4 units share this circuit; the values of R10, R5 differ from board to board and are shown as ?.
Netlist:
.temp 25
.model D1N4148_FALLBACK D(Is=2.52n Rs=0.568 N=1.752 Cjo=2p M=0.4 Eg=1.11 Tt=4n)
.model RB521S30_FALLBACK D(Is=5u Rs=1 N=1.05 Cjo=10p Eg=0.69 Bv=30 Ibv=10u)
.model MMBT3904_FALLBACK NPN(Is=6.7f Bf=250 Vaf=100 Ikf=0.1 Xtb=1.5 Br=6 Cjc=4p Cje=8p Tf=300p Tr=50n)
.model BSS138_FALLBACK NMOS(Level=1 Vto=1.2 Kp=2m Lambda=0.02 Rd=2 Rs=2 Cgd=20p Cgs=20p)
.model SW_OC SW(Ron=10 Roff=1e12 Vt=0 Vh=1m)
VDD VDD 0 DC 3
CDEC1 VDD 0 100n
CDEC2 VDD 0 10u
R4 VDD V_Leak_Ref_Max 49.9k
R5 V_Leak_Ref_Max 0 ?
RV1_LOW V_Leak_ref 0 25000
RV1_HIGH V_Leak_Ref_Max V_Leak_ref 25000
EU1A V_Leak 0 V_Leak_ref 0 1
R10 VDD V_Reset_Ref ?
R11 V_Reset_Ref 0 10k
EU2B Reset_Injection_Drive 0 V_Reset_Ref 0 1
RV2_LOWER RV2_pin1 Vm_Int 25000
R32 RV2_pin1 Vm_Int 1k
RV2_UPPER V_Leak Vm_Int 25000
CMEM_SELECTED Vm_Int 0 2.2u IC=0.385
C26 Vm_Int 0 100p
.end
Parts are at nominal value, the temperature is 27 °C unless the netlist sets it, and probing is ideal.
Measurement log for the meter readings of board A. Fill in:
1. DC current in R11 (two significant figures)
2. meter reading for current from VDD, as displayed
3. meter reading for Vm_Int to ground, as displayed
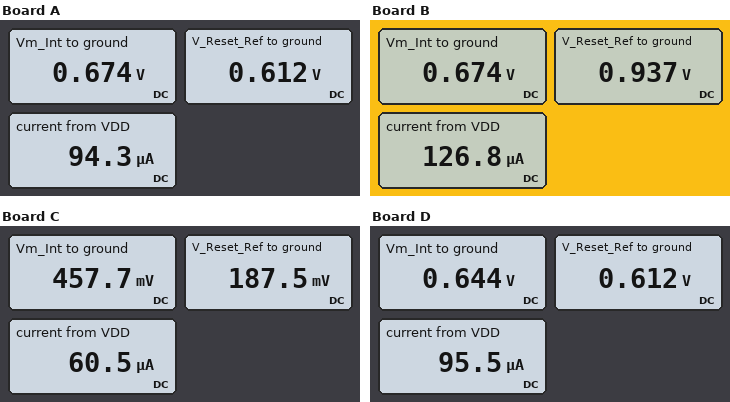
61 µA
94.3 µA
0.674 V
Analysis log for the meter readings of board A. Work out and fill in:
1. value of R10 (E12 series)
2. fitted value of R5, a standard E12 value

39 kΩ
220 kΩ
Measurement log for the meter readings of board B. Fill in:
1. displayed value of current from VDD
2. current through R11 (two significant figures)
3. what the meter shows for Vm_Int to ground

126.8 µA
94 µA
0.674 V
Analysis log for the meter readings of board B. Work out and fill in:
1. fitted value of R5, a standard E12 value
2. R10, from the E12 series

220 kΩ
22 kΩ
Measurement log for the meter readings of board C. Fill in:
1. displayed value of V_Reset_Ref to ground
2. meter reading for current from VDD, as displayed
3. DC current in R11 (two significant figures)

187.5 mV
60.5 µA
19 µA
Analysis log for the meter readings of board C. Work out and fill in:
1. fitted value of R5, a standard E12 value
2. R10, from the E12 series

39 kΩ
150 kΩ
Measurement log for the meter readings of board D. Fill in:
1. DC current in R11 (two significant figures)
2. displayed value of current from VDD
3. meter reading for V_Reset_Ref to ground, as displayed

61 µA
95.5 µA
0.612 V
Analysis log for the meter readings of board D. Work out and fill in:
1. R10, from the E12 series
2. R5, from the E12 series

39 kΩ
150 kΩ
